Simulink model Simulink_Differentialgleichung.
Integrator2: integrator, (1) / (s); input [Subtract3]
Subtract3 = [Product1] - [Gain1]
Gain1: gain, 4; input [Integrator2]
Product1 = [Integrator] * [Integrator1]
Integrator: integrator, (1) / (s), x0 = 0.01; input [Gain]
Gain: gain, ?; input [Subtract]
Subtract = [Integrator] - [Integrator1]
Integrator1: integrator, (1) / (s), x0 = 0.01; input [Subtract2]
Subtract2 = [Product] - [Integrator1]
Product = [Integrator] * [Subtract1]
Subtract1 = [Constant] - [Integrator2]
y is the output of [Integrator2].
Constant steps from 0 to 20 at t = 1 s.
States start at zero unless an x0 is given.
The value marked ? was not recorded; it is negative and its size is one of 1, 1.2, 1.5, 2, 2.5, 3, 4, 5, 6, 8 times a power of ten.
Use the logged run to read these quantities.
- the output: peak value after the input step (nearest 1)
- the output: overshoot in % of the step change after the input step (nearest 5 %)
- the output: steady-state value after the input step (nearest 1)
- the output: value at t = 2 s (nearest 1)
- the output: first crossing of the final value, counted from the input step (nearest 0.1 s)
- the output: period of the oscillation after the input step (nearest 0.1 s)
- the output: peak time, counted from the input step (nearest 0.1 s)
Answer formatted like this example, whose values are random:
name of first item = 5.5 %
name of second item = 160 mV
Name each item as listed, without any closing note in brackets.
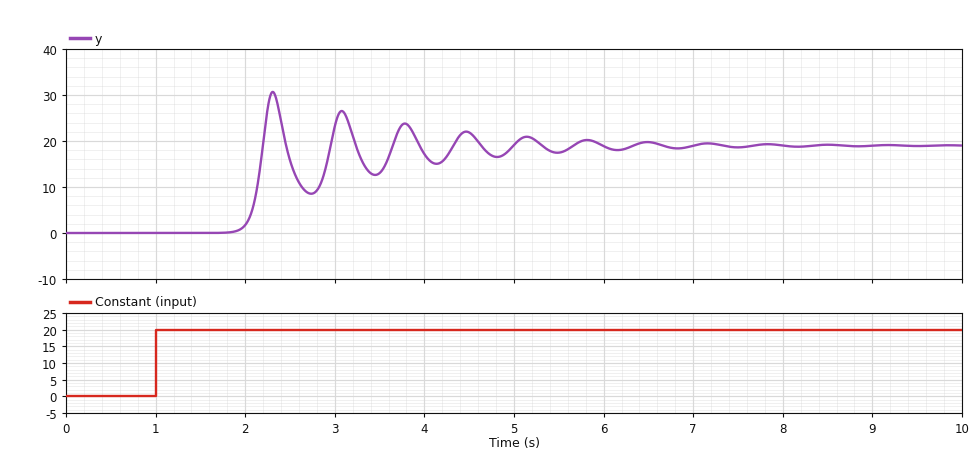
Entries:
the output: peak value after the input step = 31
the output: overshoot in % of the step change after the input step = 60 %
the output: steady-state value after the input step = 19
the output: value at t = 2 s = 2
the output: first crossing of the final value, counted from the input step = 1.2 s
the output: period of the oscillation after the input step = 0.8 s
the output: peak time, counted from the input step = 1.3 s
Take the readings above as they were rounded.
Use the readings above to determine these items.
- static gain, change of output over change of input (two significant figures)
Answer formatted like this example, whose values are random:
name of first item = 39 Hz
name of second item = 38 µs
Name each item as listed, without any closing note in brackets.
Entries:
static gain, change of output over change of input = 0.95
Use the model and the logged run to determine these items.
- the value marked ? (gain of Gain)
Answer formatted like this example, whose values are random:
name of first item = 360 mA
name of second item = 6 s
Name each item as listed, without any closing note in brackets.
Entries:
the value marked ? = -5
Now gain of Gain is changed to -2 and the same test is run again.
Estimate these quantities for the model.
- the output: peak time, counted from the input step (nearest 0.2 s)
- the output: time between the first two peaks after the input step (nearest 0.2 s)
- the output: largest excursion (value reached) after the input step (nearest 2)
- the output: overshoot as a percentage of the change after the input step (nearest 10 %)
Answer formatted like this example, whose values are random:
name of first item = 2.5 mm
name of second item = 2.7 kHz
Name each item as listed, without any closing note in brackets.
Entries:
the output: peak time, counted from the input step = 1.8 s
the output: time between the first two peaks after the input step = 0.8 s
the output: largest excursion (value reached) after the input step = 28
the output: overshoot as a percentage of the change after the input step = 50 %
